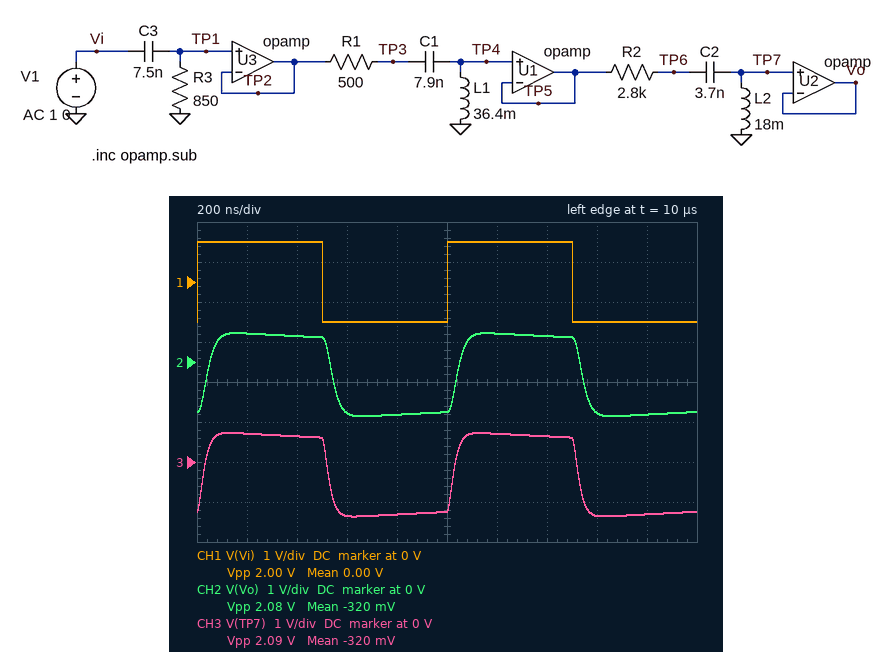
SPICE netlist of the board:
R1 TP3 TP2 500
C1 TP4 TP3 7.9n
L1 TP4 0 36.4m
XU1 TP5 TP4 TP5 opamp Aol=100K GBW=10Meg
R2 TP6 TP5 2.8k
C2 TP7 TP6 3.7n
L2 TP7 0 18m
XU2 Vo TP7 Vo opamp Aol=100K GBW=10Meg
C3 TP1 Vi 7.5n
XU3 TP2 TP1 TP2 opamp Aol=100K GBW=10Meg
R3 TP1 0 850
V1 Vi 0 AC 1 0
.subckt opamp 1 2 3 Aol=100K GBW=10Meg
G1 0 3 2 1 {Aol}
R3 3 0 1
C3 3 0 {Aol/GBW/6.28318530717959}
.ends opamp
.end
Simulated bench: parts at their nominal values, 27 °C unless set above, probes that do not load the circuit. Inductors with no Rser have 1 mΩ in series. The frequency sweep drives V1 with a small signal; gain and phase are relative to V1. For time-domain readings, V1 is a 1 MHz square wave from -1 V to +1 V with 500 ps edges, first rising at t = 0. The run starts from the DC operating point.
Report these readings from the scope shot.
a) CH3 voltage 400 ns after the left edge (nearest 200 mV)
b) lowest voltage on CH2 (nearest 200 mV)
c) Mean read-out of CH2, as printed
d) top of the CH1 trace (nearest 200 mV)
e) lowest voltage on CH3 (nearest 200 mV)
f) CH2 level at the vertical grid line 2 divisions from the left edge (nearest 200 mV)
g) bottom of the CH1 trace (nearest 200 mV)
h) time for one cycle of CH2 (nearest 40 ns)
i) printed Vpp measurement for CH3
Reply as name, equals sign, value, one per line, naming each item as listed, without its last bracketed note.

CH3 voltage 400 ns after the left edge = 600 mV
lowest voltage on CH2 = -1.4 V
Mean read-out of CH2, as printed = -320 mV
top of the CH1 trace = 1.0 V
lowest voltage on CH3 = -1.4 V
CH2 level at the vertical grid line 2 divisions from the left edge = 600 mV
bottom of the CH1 trace = -1.0 V
time for one cycle of CH2 = 1.00 µs
printed Vpp measurement for CH3 = 2.09 V
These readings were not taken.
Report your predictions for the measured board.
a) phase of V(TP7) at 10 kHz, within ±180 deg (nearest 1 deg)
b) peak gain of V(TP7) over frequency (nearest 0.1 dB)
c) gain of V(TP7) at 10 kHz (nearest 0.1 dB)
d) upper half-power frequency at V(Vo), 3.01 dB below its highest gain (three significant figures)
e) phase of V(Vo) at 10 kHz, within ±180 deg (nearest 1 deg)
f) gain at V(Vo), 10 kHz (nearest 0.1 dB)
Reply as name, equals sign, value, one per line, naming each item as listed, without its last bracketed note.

phase of V(TP7) at 10 kHz, within ±180 deg = -92 deg
peak gain of V(TP7) over frequency = 0 dB
gain of V(TP7) at 10 kHz = -8.0 dB
upper half-power frequency at V(Vo), 3.01 dB below its highest gain = 5.12 MHz
phase of V(Vo) at 10 kHz, within ±180 deg = -92 deg
gain at V(Vo), 10 kHz = -8.0 dB
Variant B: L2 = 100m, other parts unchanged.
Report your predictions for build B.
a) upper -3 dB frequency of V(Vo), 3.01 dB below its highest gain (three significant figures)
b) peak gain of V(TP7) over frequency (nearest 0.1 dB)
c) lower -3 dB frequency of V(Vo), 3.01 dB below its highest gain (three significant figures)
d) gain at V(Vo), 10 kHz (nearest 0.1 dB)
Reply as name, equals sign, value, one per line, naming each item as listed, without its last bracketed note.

upper -3 dB frequency of V(Vo), 3.01 dB below its highest gain = 10.9 kHz
peak gain of V(TP7) over frequency = 9.3 dB
lower -3 dB frequency of V(Vo), 3.01 dB below its highest gain = 8.67 kHz
gain at V(Vo), 10 kHz = 8.7 dB
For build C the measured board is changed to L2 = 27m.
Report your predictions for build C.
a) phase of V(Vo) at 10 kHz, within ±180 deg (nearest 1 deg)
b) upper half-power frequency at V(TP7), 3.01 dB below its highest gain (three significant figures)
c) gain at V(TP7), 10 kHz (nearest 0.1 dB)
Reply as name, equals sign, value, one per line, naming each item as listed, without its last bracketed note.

phase of V(Vo) at 10 kHz, within ±180 deg = -98 deg
upper half-power frequency at V(TP7), 3.01 dB below its highest gain = 6.46 MHz
gain at V(TP7), 10 kHz = -3.6 dB
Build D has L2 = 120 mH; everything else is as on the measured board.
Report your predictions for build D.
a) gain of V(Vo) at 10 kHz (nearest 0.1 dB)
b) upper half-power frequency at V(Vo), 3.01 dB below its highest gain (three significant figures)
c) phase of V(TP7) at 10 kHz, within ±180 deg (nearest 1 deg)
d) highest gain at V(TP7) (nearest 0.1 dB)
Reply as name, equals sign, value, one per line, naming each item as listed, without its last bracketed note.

gain of V(Vo) at 10 kHz = 8.4 dB
upper half-power frequency at V(Vo), 3.01 dB below its highest gain = 10.8 kHz
phase of V(TP7) at 10 kHz, within ±180 deg = 170 deg
highest gain at V(TP7) = 9.1 dB
